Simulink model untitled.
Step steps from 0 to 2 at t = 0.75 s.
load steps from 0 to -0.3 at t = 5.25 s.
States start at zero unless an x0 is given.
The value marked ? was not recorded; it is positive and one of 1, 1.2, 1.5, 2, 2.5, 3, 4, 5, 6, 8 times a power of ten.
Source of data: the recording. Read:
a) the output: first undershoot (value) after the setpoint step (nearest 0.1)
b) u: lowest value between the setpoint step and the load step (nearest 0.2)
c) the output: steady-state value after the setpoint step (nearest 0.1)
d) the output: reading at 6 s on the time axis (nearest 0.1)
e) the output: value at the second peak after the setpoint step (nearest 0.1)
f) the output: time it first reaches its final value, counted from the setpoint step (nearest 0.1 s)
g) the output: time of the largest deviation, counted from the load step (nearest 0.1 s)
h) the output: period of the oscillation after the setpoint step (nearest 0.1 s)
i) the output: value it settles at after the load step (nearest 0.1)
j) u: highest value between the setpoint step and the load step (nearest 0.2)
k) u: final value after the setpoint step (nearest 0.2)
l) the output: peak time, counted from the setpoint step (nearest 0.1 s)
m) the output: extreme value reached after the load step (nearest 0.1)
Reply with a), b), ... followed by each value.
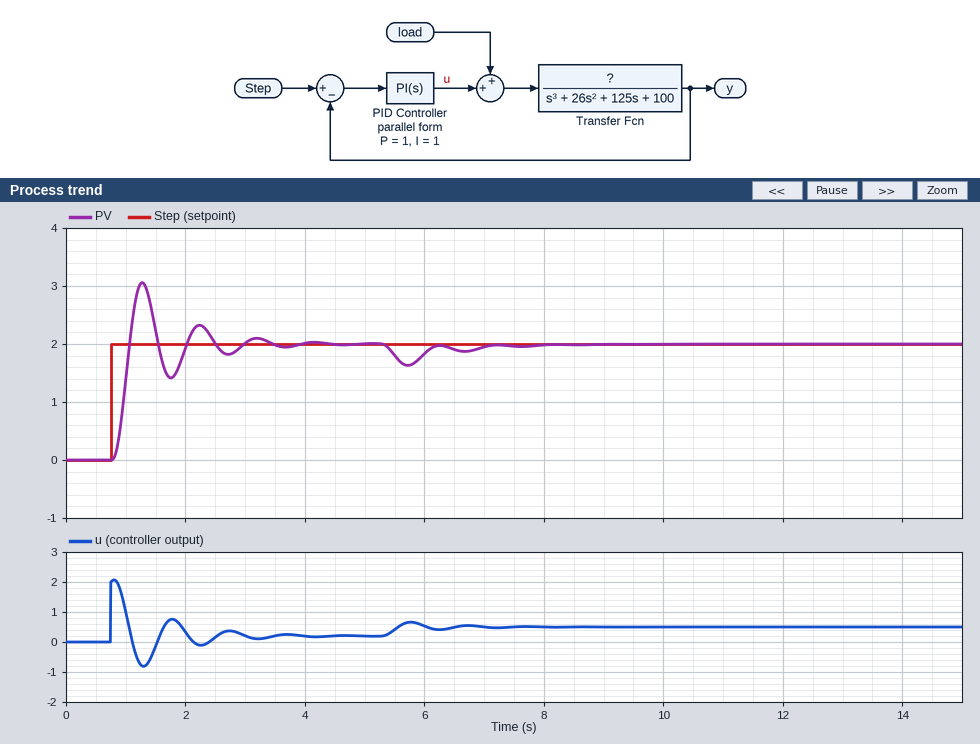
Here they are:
a) 1.4
b) -0.8
c) 2.0
d) 1.8
e) 2.3
f) 0.3 s
g) 0.5 s
h) 1.0 s
i) 2.0
j) 2.0
k) 0.2
l) 0.5 s
m) 1.6
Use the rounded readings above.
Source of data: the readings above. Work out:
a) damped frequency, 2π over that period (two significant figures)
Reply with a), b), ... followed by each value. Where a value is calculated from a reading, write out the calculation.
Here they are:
a) 2π / 1 = 6.3 rad/s
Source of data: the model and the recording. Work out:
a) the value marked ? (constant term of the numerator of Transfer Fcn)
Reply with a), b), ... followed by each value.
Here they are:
a) 1000
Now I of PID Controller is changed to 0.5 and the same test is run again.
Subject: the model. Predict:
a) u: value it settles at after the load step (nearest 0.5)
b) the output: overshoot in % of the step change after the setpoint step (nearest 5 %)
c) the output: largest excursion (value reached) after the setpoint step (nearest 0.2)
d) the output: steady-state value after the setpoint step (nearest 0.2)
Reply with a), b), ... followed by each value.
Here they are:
a) 0.5
b) 40 %
c) 2.8
d) 2.0
